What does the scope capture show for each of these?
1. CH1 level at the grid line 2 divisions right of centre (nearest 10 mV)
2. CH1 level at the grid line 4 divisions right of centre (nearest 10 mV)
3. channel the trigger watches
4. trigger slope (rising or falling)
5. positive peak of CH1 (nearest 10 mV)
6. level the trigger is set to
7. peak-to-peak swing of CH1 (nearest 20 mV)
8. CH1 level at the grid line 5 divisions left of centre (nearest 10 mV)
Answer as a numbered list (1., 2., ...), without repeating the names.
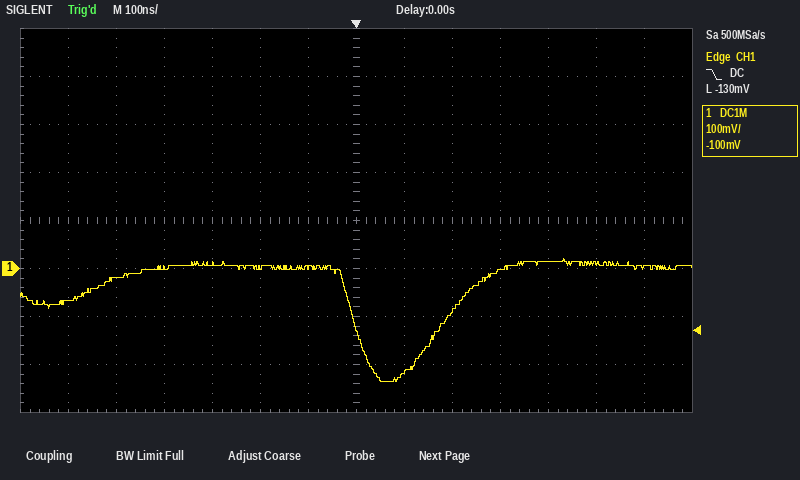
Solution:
1. -90 mV
2. 10 mV
3. CH1
4. falling
5. 20 mV
6. -130 mV
7. 260 mV
8. -20 mV
